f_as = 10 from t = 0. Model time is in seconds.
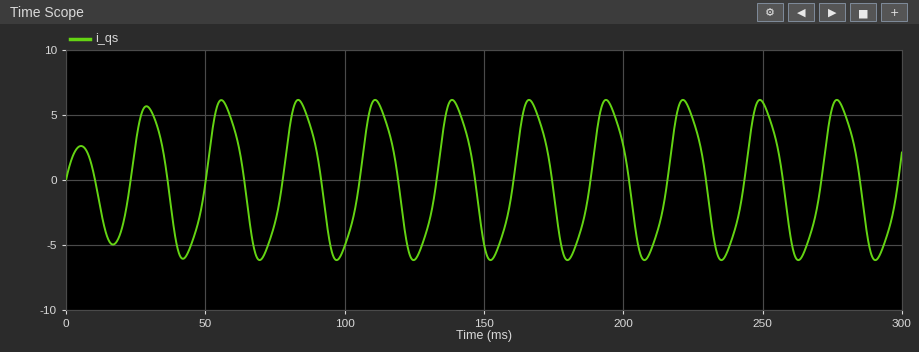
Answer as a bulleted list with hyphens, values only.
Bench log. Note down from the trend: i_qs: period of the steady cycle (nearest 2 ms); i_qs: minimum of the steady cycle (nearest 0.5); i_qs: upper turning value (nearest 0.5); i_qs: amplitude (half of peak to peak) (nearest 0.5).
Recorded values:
- 28 ms
- -6.0
- 6.0
- 6.0
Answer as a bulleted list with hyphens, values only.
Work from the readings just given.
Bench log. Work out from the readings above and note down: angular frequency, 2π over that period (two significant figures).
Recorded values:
- 0.22 rad/ms
